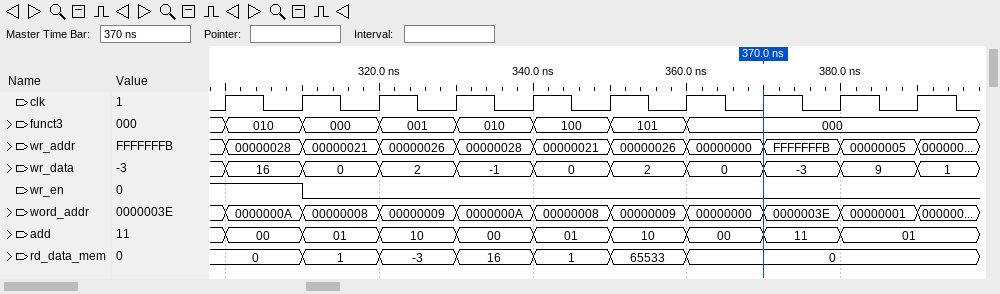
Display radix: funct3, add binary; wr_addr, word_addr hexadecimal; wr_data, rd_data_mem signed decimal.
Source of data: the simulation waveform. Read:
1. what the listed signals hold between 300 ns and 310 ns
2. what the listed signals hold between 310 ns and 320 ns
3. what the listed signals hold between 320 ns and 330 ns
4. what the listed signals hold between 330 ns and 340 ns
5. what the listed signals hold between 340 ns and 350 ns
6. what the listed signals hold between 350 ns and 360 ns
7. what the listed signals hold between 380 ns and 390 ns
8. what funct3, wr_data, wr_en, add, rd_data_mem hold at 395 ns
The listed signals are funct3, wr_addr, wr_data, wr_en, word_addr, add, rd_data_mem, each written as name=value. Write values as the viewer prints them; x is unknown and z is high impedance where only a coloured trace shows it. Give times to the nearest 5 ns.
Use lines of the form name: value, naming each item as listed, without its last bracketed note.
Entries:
what the listed signals hold between 300 ns and 310 ns: funct3=010, wr_addr=00000028, wr_data=16, wr_en=1, word_addr=0000000A, add=00, rd_data_mem=0
what the listed signals hold between 310 ns and 320 ns: funct3=000, wr_addr=00000021, wr_data=0, wr_en=0, word_addr=00000008, add=01, rd_data_mem=1
what the listed signals hold between 320 ns and 330 ns: funct3=001, wr_addr=00000026, wr_data=2, wr_en=0, word_addr=00000009, add=10, rd_data_mem=-3
what the listed signals hold between 330 ns and 340 ns: funct3=010, wr_addr=00000028, wr_data=-1, wr_en=0, word_addr=0000000A, add=00, rd_data_mem=16
what the listed signals hold between 340 ns and 350 ns: funct3=100, wr_addr=00000021, wr_data=0, wr_en=0, word_addr=00000008, add=01, rd_data_mem=1
what the listed signals hold between 350 ns and 360 ns: funct3=101, wr_addr=00000026, wr_data=2, wr_en=0, word_addr=00000009, add=10, rd_data_mem=65533
what the listed signals hold between 380 ns and 390 ns: funct3=000, wr_addr=00000005, wr_data=9, wr_en=0, word_addr=00000001, add=01, rd_data_mem=0
what funct3, wr_data, wr_en, add, rd_data_mem hold at 395 ns: funct3=000, wr_data=1, wr_en=0, add=01, rd_data_mem=0
